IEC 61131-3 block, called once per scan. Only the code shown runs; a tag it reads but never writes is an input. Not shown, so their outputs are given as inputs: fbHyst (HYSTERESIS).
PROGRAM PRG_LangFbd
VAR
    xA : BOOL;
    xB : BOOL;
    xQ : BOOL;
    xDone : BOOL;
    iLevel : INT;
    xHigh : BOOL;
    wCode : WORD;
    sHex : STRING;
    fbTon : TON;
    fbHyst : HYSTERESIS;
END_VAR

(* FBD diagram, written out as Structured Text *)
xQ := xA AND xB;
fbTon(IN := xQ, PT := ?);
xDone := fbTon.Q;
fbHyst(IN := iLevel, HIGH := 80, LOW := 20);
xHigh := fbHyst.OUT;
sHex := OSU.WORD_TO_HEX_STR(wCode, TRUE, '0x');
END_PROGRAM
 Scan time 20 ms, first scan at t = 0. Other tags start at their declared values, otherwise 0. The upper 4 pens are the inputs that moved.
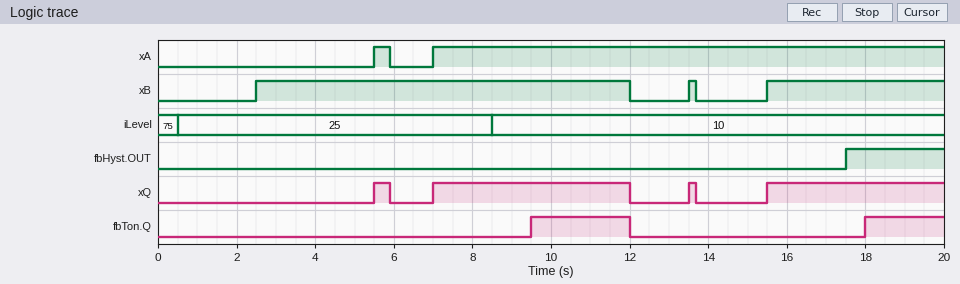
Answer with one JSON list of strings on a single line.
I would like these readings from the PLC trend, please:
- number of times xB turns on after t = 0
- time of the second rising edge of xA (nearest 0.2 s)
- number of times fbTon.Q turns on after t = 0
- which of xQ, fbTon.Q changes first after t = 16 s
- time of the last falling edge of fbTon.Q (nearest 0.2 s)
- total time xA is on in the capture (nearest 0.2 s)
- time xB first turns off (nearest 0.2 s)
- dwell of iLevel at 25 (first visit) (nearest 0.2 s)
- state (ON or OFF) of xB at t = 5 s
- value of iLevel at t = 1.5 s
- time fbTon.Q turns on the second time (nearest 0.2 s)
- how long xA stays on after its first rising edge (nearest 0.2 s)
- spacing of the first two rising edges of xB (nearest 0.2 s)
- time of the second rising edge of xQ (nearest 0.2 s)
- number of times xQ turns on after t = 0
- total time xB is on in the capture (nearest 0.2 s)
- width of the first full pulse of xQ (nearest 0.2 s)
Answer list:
["3", "7.0 s", "2", "fbTon.Q", "12.0 s", "13.4 s", "12.0 s", "8.0 s", "ON", "25", "18.0 s", "0.4 s", "11.0 s", "7.0 s", "4", "14.2 s", "0.4 s"]
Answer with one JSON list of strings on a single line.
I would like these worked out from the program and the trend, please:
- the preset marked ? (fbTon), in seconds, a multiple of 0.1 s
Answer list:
["2.5 s"]
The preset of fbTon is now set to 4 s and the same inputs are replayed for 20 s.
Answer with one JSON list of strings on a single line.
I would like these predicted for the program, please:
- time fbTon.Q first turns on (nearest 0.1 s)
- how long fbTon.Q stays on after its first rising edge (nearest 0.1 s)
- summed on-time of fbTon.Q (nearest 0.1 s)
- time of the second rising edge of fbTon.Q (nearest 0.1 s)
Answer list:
["11.0 s", "1.0 s", "1.5 s", "19.5 s"]
